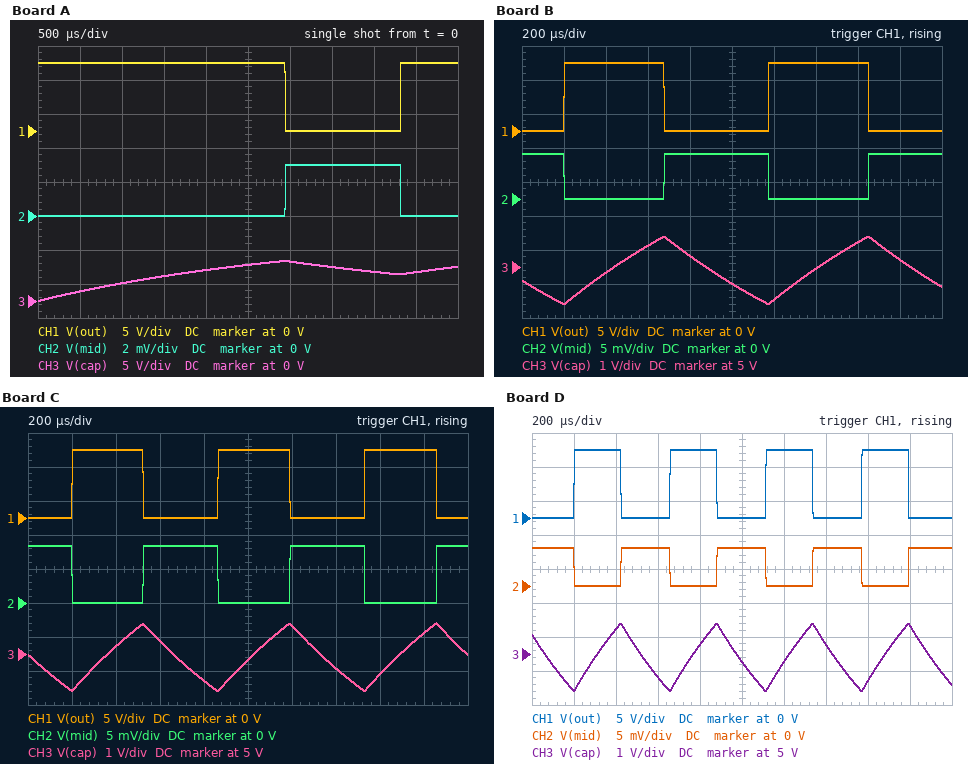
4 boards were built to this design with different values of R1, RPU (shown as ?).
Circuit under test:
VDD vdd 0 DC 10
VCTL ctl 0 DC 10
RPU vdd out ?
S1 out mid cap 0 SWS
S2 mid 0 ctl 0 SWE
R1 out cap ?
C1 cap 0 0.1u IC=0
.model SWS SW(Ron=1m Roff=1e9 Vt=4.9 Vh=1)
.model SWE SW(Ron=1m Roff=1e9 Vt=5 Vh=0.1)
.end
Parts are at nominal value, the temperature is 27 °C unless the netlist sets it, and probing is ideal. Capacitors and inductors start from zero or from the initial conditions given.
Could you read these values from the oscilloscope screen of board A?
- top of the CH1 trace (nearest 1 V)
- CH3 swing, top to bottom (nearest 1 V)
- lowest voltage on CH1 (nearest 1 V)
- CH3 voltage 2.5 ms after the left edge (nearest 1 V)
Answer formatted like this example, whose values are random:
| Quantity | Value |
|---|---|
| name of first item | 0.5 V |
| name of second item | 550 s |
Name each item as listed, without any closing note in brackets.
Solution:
| Quantity | Value |
|---|---|
| top of the CH1 trace | 10 V |
| CH3 swing, top to bottom | 6 V |
| lowest voltage on CH1 | 0 V |
| CH3 voltage 2.5 ms after the left edge | 5 V |
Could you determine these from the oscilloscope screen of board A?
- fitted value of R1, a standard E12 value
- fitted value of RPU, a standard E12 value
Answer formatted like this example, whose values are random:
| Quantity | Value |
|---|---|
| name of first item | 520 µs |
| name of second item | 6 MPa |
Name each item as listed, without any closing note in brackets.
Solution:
| Quantity | Value |
|---|---|
| fitted value of R1, a standard E12 value | 33 kΩ |
| fitted value of RPU, a standard E12 value | 3.3 Ω |
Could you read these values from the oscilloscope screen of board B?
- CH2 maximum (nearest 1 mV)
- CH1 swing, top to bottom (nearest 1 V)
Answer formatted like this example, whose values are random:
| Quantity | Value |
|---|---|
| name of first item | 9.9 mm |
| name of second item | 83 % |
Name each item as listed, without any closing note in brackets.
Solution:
| Quantity | Value |
|---|---|
| CH2 maximum | 7 mV |
| CH1 swing, top to bottom | 10 V |
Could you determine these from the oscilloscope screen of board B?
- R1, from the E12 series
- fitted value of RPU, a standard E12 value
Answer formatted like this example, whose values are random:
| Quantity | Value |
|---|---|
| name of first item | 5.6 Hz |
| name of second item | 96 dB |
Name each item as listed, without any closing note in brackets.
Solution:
| Quantity | Value |
|---|---|
| R1, from the E12 series | 12 kΩ |
| fitted value of RPU, a standard E12 value | 1.5 Ω |
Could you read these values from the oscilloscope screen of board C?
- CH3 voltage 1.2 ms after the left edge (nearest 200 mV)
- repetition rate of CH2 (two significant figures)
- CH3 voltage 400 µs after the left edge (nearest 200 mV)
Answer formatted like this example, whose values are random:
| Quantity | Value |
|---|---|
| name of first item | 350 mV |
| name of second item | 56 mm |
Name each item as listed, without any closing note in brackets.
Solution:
| Quantity | Value |
|---|---|
| CH3 voltage 1.2 ms after the left edge | 5.8 V |
| repetition rate of CH2 | 1.5 kHz |
| CH3 voltage 400 µs after the left edge | 5.2 V |
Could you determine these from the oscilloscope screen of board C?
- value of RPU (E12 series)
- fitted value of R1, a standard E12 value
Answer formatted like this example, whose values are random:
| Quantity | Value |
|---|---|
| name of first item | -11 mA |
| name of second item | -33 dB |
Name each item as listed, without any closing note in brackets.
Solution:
| Quantity | Value |
|---|---|
| value of RPU | 1.2 Ω |
| fitted value of R1, a standard E12 value | 8.2 kΩ |
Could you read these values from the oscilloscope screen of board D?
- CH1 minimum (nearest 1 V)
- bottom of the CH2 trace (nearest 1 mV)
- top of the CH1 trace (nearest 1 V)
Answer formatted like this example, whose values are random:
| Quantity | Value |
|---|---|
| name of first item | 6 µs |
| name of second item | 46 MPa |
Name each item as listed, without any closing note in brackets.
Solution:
| Quantity | Value |
|---|---|
| CH1 minimum | 0 V |
| bottom of the CH2 trace | 0 V |
| top of the CH1 trace | 10 V |
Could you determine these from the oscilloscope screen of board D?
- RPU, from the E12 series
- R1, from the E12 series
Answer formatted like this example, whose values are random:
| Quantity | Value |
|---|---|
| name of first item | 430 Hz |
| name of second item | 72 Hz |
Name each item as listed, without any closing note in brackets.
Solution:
| Quantity | Value |
|---|---|
| RPU, from the E12 series | 1.8 Ω |
| R1, from the E12 series | 5.6 kΩ |
